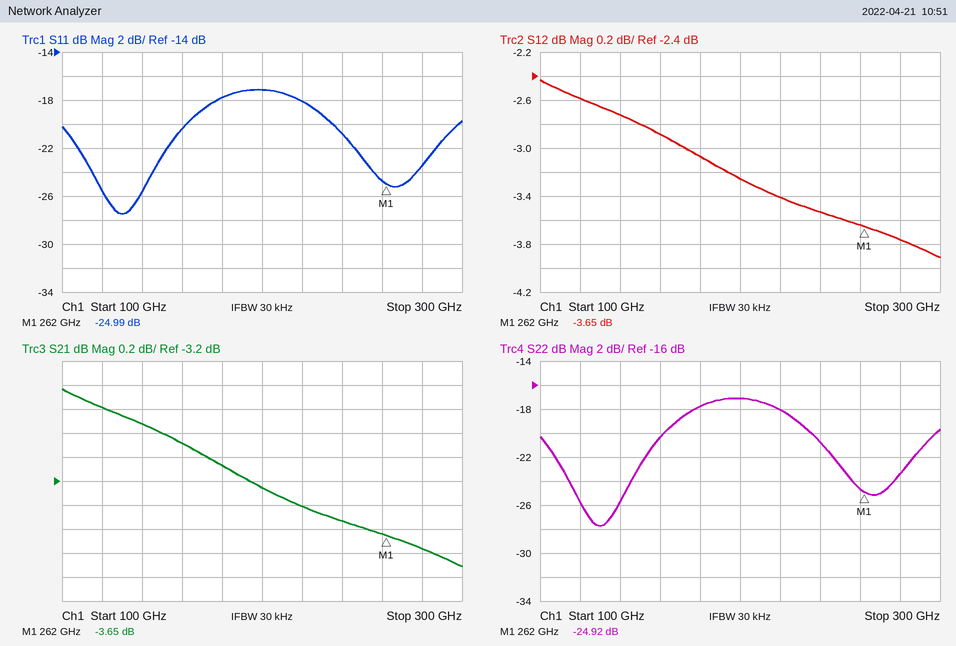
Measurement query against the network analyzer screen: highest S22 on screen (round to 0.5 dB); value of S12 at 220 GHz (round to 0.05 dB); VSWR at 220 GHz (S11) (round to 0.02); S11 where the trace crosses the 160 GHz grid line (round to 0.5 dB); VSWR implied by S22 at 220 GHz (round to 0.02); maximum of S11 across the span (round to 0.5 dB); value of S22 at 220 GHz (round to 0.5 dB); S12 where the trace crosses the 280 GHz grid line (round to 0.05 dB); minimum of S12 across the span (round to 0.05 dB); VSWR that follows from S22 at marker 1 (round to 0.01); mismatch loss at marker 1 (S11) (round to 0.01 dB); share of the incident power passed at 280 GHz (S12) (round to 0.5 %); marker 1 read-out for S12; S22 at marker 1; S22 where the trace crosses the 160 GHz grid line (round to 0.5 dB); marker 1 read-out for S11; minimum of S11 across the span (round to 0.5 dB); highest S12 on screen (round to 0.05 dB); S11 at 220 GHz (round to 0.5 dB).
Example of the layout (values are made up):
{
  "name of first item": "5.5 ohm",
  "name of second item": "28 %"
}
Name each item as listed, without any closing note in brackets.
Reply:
{
  "highest S22 on screen": "-17.0 dB",
  "value of S12 at 220 GHz": "-3.40 dB",
  "VSWR at 220 GHz (S11)": "1.28",
  "S11 where the trace crosses the 160 GHz grid line": "-20.5 dB",
  "VSWR implied by S22 at 220 GHz": "1.28",
  "maximum of S11 across the span": "-17.0 dB",
  "value of S22 at 220 GHz": "-18.0 dB",
  "S12 where the trace crosses the 280 GHz grid line": "-3.75 dB",
  "minimum of S12 across the span": "-3.90 dB",
  "VSWR that follows from S22 at marker 1": "1.12",
  "mismatch loss at marker 1 (S11)": "0.01 dB",
  "share of the incident power passed at 280 GHz (S12)": "42.0 %",
  "marker 1 read-out for S12": "-3.65 dB",
  "S22 at marker 1": "-24.92 dB",
  "S22 where the trace crosses the 160 GHz grid line": "-20.5 dB",
  "marker 1 read-out for S11": "-24.99 dB",
  "minimum of S11 across the span": "-27.5 dB",
  "highest S12 on screen": "-2.45 dB",
  "S11 at 220 GHz": "-18.0 dB"
}
